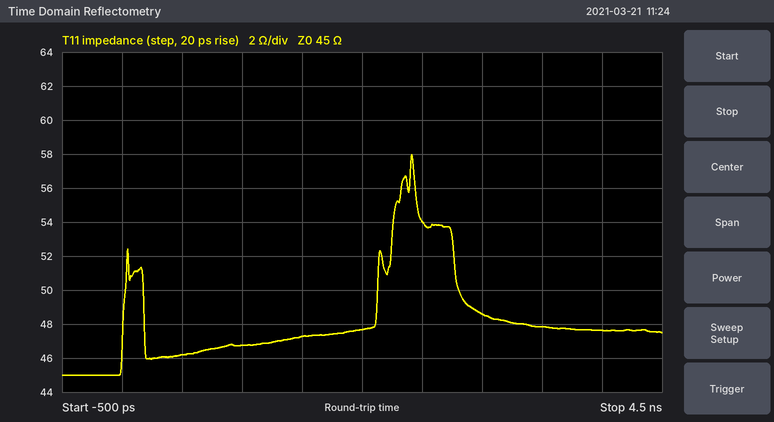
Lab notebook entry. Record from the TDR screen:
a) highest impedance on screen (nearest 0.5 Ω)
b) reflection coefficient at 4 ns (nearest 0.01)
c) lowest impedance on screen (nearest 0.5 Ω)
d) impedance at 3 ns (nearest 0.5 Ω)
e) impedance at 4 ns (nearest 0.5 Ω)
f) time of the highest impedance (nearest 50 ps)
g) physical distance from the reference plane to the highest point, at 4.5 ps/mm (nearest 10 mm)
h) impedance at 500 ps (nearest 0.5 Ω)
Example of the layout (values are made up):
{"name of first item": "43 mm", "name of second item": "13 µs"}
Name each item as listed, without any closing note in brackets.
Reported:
{"highest impedance on screen": "58.0 Ω", "reflection coefficient at 4 ns": "+0.03", "lowest impedance on screen": "45.0 Ω", "impedance at 3 ns": "48.5 Ω", "impedance at 4 ns": "47.5 Ω", "time of the highest impedance": "2.40 ns", "physical distance from the reference plane to the highest point, at 4.5 ps/mm": "270 mm", "impedance at 500 ps": "46.0 Ω"}
